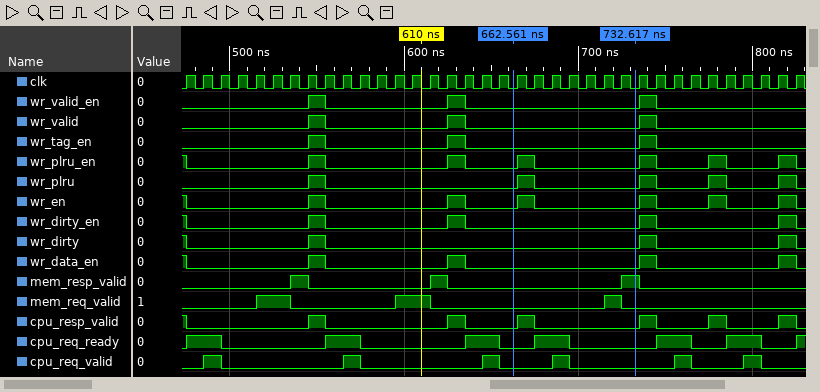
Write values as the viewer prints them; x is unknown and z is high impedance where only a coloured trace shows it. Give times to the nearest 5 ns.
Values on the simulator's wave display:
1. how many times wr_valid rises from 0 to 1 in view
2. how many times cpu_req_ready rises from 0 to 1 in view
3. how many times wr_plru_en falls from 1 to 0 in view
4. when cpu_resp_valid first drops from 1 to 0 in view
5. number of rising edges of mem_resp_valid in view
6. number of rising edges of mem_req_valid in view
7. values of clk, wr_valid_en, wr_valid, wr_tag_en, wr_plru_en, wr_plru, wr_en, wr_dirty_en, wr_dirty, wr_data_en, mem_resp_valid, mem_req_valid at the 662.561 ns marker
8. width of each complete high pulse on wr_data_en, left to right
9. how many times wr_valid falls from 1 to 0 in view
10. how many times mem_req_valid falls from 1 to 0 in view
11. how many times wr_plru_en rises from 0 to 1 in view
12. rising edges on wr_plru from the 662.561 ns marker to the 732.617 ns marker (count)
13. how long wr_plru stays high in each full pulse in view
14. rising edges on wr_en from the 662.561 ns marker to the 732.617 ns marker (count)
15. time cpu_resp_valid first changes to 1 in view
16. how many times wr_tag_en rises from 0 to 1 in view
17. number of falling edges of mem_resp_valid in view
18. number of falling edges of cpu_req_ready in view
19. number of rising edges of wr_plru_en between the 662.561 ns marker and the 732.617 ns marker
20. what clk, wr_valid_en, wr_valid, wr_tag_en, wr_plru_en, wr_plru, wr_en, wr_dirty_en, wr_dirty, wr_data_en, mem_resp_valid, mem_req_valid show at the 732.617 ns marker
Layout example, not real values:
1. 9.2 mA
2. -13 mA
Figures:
1. 3
2. 7
3. 7
4. 475 ns
5. 3
6. 3
7. clk=0, wr_valid_en=0, wr_valid=0, wr_tag_en=0, wr_plru_en=0, wr_plru=0, wr_en=0, wr_dirty_en=0, wr_dirty=0, wr_data_en=0, mem_resp_valid=0, mem_req_valid=0
8. 10 ns, 10 ns, 10 ns, 10 ns
9. 3
10. 3
11. 6
12. 1
13. 10 ns, 10 ns, 10 ns, 10 ns, 10 ns
14. 1
15. 545 ns
16. 3
17. 3
18. 6
19. 1
20. clk=0, wr_valid_en=0, wr_valid=0, wr_tag_en=0, wr_plru_en=0, wr_plru=0, wr_en=0, wr_dirty_en=0, wr_dirty=0, wr_data_en=0, mem_resp_valid=1, mem_req_valid=0
